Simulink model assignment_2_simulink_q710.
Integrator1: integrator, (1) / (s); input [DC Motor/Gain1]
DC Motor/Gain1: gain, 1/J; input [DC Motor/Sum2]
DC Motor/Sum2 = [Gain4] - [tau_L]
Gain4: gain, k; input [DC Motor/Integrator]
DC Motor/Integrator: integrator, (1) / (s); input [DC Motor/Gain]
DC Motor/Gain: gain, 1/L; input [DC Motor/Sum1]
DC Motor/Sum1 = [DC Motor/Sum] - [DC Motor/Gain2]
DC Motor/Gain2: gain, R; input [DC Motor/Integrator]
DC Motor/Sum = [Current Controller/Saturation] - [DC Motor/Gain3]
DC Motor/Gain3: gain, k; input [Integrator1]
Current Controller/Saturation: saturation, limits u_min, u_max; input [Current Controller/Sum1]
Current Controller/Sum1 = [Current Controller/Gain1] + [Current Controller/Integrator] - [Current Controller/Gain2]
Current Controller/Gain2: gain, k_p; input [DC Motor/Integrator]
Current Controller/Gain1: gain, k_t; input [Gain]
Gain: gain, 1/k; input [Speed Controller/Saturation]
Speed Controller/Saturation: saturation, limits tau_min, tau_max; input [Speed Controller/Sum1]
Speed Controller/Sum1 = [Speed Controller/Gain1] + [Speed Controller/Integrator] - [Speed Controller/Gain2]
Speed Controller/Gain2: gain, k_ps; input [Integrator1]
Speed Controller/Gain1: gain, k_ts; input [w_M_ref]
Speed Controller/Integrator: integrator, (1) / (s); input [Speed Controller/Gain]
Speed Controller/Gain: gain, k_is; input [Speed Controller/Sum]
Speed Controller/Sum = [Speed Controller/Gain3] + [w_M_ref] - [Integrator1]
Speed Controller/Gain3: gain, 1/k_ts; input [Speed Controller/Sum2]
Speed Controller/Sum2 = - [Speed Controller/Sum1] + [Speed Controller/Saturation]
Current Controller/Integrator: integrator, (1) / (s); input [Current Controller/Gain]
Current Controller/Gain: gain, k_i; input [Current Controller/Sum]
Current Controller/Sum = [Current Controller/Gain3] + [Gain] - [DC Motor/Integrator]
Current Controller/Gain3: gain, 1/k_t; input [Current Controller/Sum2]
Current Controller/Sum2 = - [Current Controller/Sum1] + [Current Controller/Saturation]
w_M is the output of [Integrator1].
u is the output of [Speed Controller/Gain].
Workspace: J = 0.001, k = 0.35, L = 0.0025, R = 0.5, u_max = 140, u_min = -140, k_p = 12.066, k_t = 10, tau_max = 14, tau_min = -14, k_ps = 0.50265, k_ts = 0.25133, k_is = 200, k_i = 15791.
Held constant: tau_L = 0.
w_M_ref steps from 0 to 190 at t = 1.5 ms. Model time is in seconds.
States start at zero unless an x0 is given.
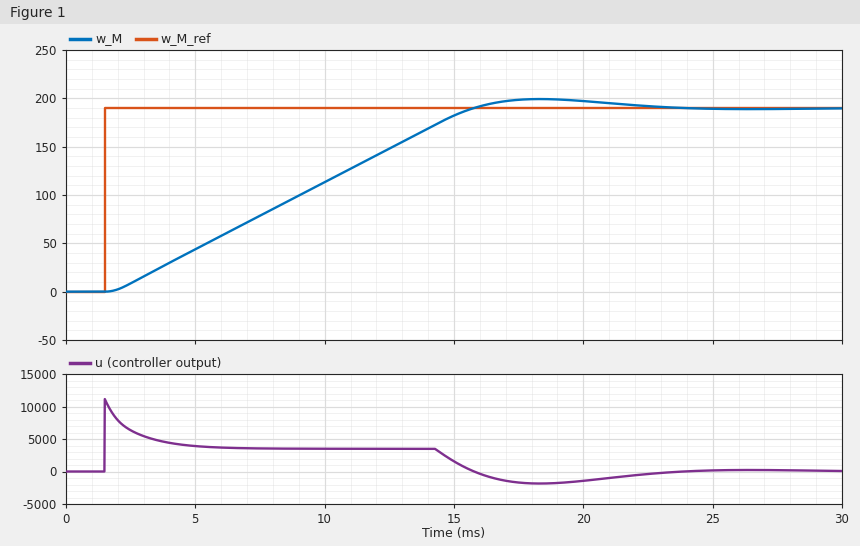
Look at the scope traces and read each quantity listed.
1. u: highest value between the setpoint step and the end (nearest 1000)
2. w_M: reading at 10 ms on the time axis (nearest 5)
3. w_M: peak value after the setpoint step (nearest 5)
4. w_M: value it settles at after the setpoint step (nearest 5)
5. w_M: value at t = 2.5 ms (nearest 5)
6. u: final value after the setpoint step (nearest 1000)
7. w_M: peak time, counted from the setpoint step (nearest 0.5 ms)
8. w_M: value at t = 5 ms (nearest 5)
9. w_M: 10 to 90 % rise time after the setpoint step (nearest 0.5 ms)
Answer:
11000
115
200
190
10
0
17.0 ms
45
11.0 ms
